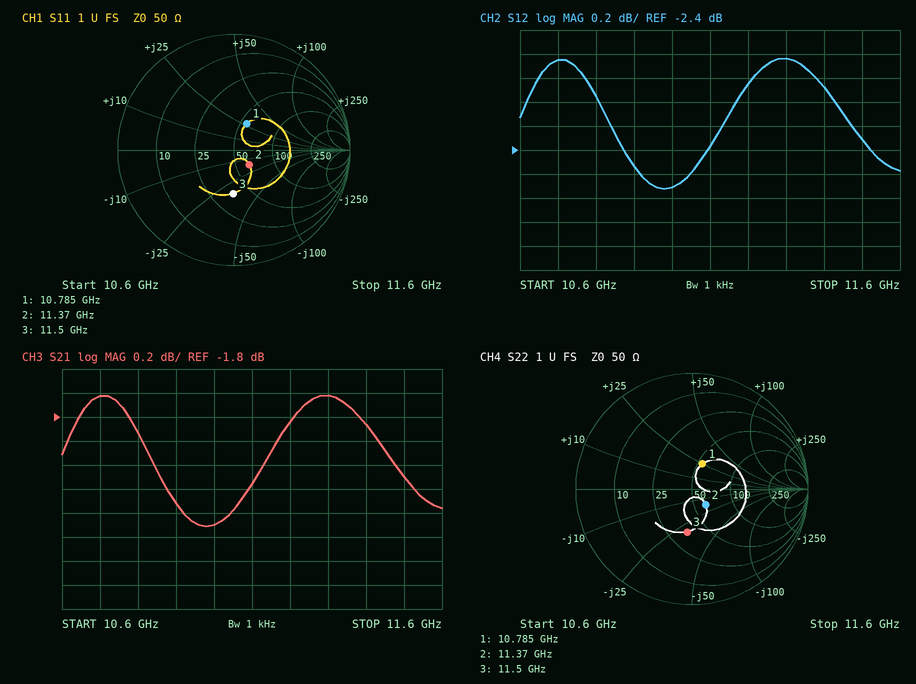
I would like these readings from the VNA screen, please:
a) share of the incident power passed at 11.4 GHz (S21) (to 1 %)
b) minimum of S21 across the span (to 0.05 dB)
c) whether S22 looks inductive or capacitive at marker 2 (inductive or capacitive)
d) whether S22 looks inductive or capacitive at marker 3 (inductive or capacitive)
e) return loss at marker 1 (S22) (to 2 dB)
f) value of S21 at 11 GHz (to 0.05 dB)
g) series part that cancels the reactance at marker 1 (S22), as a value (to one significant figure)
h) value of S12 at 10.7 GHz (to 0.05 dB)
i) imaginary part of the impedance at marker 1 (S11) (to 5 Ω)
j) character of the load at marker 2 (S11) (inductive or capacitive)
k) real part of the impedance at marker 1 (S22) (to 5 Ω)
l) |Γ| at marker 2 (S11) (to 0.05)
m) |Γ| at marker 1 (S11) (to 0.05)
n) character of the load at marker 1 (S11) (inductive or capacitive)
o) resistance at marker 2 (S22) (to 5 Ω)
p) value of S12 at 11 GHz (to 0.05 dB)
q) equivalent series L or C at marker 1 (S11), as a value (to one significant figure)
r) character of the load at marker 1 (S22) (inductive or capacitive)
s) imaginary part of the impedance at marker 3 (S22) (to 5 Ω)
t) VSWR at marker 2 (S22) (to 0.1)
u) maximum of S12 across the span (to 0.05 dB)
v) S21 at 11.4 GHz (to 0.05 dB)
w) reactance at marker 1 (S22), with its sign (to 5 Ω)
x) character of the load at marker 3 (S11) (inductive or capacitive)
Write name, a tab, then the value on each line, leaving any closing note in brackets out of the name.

share of the incident power passed at 11.4 GHz (S21)	65 %
minimum of S21 across the span	-2.70 dB
whether S22 looks inductive or capacitive at marker 2	capacitive
whether S22 looks inductive or capacitive at marker 3	capacitive
return loss at marker 1 (S22)	12 dB
value of S21 at 11 GHz	-2.70 dB
series part that cancels the reactance at marker 1 (S22), as a value	600 fF
value of S12 at 10.7 GHz	-1.65 dB
imaginary part of the impedance at marker 1 (S11)	+25 Ω
character of the load at marker 2 (S11)	capacitive
real part of the impedance at marker 1 (S22)	55 Ω
|Γ| at marker 2 (S11)	0.20
|Γ| at marker 1 (S11)	0.25
character of the load at marker 1 (S11)	inductive
resistance at marker 2 (S22)	60 Ω
value of S12 at 11 GHz	-2.70 dB
equivalent series L or C at marker 1 (S11), as a value	400 pH
character of the load at marker 1 (S22)	inductive
imaginary part of the impedance at marker 3 (S22)	-30 Ω
VSWR at marker 2 (S22)	1.4
maximum of S12 across the span	-1.65 dB
S21 at 11.4 GHz	-1.85 dB
reactance at marker 1 (S22), with its sign	+25 Ω
character of the load at marker 3 (S11)	capacitive
